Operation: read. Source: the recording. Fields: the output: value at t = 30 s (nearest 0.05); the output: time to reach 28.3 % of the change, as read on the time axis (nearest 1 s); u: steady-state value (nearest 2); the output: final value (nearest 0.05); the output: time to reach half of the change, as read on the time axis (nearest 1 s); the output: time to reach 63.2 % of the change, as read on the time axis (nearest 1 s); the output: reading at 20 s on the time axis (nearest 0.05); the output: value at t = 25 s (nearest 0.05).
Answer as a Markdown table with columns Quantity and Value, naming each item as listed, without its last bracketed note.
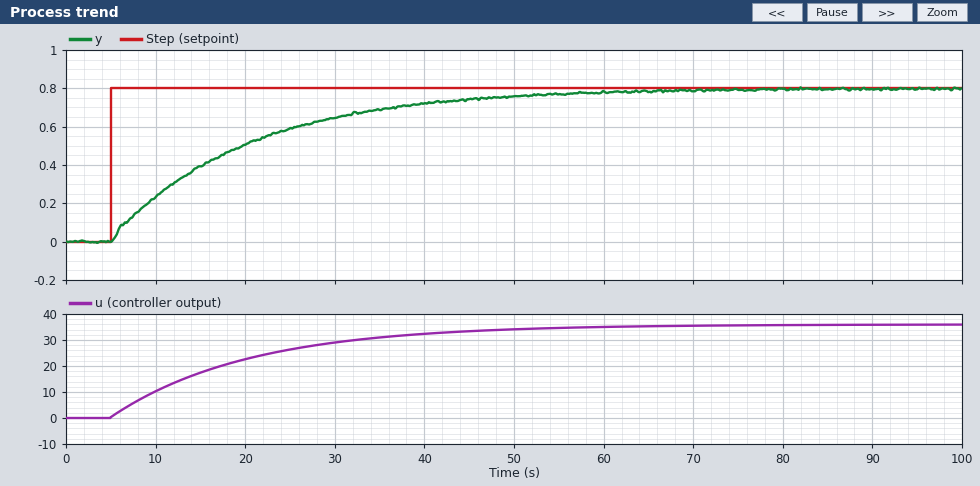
| Quantity | Value |
|---|---|
| the output: value at t = 30 s | 0.65 |
| the output: time to reach 28.3 % of the change, as read on the time axis | 10 s |
| u: steady-state value | 36 |
| the output: final value | 0.80 |
| the output: time to reach half of the change, as read on the time axis | 15 s |
| the output: time to reach 63.2 % of the change, as read on the time axis | 20 s |
| the output: reading at 20 s on the time axis | 0.50 |
| the output: value at t = 25 s | 0.60 |
